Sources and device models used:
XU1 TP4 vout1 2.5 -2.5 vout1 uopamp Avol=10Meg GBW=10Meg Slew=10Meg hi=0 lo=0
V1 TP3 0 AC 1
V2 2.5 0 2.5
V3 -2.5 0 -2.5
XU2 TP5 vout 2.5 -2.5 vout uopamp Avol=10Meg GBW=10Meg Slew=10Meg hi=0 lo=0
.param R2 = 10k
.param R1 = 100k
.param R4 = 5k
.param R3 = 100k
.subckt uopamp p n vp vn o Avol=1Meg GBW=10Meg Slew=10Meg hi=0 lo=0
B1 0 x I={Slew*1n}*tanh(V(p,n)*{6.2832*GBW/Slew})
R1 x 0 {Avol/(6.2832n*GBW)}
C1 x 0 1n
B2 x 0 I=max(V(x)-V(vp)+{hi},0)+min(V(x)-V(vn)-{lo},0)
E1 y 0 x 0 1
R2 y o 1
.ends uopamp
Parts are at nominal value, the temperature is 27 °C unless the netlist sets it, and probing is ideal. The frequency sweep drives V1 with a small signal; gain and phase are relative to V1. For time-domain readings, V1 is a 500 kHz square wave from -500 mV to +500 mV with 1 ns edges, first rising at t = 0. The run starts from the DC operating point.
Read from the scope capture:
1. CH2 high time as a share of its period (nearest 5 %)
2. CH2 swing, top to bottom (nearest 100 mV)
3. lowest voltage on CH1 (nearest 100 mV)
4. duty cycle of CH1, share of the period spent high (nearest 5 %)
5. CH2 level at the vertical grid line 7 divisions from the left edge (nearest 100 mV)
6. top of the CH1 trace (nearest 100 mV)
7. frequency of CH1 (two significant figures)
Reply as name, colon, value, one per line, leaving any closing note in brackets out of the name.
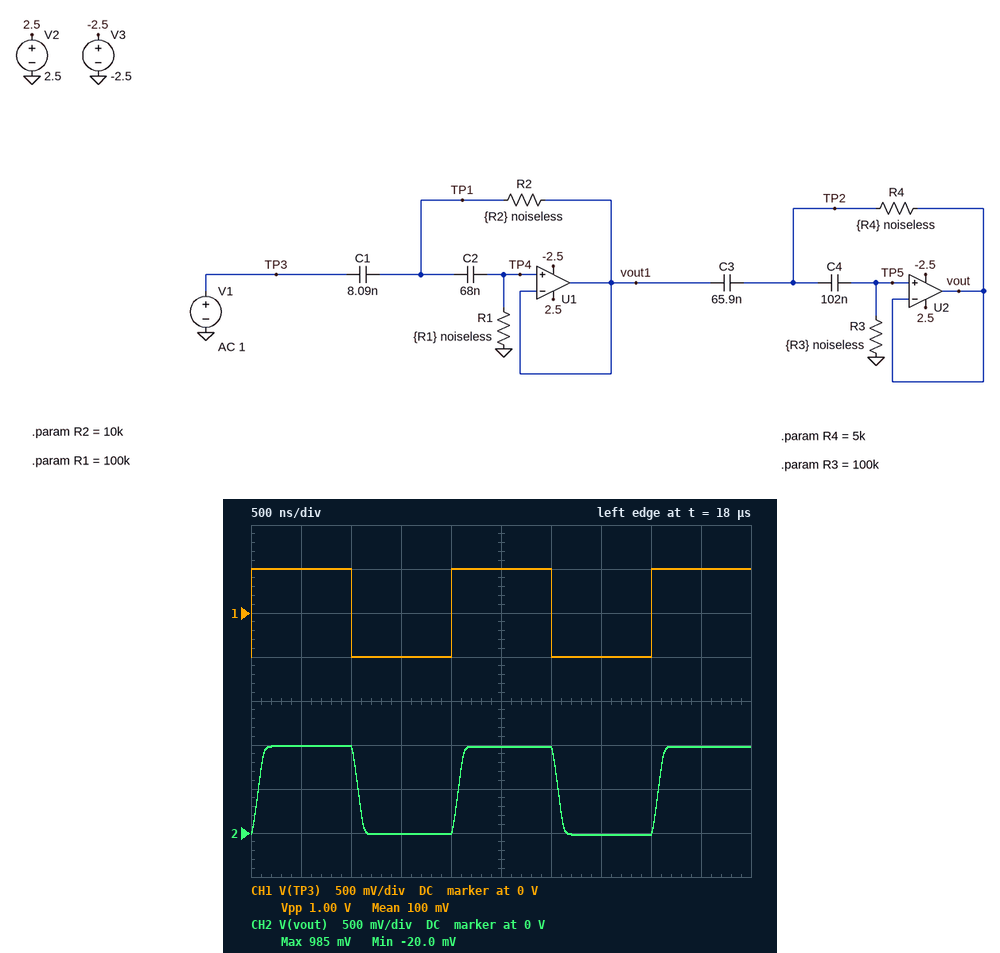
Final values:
CH2 high time as a share of its period: 50 %
CH2 swing, top to bottom: 1.0 V
lowest voltage on CH1: -500 mV
duty cycle of CH1, share of the period spent high: 50 %
CH2 level at the vertical grid line 7 divisions from the left edge: 0 V
top of the CH1 trace: 500 mV
frequency of CH1: 500 kHz
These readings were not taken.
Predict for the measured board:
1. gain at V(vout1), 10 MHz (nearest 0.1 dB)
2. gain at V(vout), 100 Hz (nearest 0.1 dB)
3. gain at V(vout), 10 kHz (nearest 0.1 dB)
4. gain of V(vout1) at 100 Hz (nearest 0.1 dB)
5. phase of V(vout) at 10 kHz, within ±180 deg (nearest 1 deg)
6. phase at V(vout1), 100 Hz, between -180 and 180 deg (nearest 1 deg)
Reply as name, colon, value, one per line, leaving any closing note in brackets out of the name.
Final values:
gain at V(vout1), 10 MHz: -3.0 dB
gain at V(vout), 100 Hz: -5.9 dB
gain at V(vout), 10 kHz: 0 dB
gain of V(vout1) at 100 Hz: -12.5 dB
phase of V(vout) at 10 kHz, within ±180 deg: 1 deg
phase at V(vout1), 100 Hz, between -180 and 180 deg: 149 deg
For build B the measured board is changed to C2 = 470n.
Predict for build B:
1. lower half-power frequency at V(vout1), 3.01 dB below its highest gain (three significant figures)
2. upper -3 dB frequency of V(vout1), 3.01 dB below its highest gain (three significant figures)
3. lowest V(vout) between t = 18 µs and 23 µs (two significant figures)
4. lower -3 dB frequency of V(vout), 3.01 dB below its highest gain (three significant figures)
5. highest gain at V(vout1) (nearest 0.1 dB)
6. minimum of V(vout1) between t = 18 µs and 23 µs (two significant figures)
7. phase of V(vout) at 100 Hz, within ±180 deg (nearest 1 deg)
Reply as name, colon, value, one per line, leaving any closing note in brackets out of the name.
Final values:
lower half-power frequency at V(vout1), 3.01 dB below its highest gain: 168 Hz
upper -3 dB frequency of V(vout1), 3.01 dB below its highest gain: 10.0 MHz
lowest V(vout) between t = 18 µs and 23 µs: -16 mV
lower -3 dB frequency of V(vout), 3.01 dB below its highest gain: 79.6 Hz
highest gain at V(vout1): 0 dB
minimum of V(vout1) between t = 18 µs and 23 µs: -14 mV
phase of V(vout) at 100 Hz, within ±180 deg: 139 deg
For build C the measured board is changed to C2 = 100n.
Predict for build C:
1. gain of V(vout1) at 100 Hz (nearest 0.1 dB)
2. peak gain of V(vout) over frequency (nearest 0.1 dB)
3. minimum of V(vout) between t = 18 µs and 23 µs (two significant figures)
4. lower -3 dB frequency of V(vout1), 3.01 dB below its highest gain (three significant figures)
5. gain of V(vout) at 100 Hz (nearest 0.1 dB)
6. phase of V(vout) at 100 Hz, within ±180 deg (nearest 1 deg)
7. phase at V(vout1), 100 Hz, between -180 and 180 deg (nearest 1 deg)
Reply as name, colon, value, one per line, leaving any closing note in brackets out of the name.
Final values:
gain of V(vout1) at 100 Hz: -9.6 dB
peak gain of V(vout) over frequency: 1.1 dB
minimum of V(vout) between t = 18 µs and 23 µs: -17 mV
lower -3 dB frequency of V(vout1), 3.01 dB below its highest gain: 159 Hz
gain of V(vout) at 100 Hz: -3.0 dB
phase of V(vout) at 100 Hz, within ±180 deg: -167 deg
phase at V(vout1), 100 Hz, between -180 and 180 deg: 135 deg
